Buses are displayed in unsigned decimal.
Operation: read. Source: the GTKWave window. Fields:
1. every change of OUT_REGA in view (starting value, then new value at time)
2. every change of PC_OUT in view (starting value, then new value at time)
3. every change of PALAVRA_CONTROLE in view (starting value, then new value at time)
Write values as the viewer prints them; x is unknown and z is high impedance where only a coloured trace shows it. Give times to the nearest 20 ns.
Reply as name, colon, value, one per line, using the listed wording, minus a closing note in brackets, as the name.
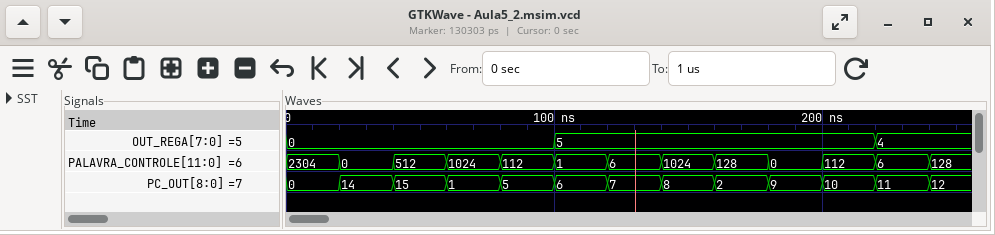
every change of OUT_REGA in view: 0, 5 at 100 ns, 4 at 220 ns
every change of PC_OUT in view: 0, 14 at 20 ns, 15 at 40 ns, 1 at 60 ns, 5 at 80 ns, 6 at 100 ns, 7 at 120 ns, 8 at 140 ns, 2 at 160 ns, 9 at 180 ns, 10 at 200 ns, 11 at 220 ns, 12 at 240 ns
every change of PALAVRA_CONTROLE in view: 2304, 0 at 20 ns, 512 at 40 ns, 1024 at 60 ns, 112 at 80 ns, 1 at 100 ns, 6 at 120 ns, 1024 at 140 ns, 128 at 160 ns, 0 at 180 ns, 112 at 200 ns, 6 at 220 ns, 128 at 240 ns
